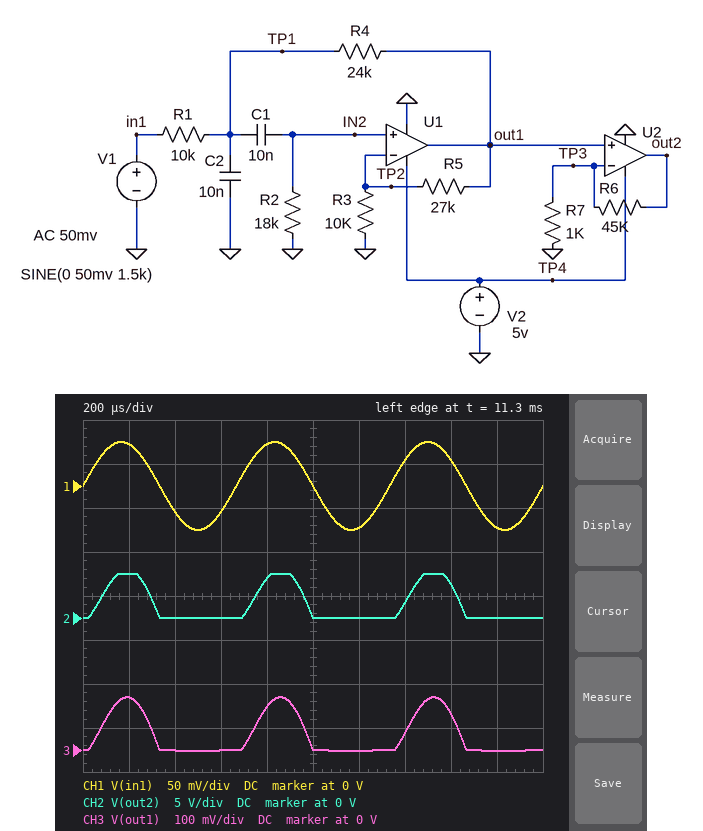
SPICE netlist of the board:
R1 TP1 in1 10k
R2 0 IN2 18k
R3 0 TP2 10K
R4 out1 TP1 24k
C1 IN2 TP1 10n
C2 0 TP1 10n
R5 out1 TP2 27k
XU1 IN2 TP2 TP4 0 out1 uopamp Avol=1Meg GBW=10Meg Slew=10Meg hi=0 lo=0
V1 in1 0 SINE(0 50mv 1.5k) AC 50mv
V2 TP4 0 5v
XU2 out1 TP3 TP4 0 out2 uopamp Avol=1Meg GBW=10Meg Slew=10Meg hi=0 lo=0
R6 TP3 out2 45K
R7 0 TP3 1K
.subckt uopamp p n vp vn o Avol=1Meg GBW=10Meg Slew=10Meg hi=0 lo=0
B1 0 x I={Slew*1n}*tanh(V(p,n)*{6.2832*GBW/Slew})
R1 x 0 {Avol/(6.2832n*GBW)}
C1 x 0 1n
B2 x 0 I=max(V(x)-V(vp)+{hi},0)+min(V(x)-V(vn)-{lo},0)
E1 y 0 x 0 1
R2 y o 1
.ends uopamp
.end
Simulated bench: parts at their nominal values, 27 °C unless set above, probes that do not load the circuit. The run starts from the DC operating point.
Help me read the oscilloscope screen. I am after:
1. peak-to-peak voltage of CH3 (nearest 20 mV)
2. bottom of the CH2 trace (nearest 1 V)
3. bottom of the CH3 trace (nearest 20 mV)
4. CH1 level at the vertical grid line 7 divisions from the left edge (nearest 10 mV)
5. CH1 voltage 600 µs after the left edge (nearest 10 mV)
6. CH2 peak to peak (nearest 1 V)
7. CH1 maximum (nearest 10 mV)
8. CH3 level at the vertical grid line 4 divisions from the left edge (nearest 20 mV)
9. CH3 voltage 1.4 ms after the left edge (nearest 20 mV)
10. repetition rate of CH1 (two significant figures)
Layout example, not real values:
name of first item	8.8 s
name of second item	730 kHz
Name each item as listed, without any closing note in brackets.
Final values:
peak-to-peak voltage of CH3	120 mV
bottom of the CH2 trace	0 V
bottom of the CH3 trace	0 V
CH1 level at the vertical grid line 7 divisions from the left edge	30 mV
CH1 voltage 600 µs after the left edge	-30 mV
CH2 peak to peak	5 V
CH1 maximum	50 mV
CH3 level at the vertical grid line 4 divisions from the left edge	100 mV
CH3 voltage 1.4 ms after the left edge	40 mV
repetition rate of CH1	1.5 kHz
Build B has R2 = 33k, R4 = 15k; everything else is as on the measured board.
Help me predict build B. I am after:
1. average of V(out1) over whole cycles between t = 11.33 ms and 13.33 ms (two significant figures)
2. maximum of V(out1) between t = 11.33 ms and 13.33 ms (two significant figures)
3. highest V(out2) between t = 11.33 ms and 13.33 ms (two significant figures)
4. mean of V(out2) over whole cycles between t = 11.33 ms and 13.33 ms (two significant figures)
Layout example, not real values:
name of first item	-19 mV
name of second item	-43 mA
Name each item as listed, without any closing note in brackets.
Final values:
average of V(out1) over whole cycles between t = 11.33 ms and 13.33 ms	51 mV
maximum of V(out1) between t = 11.33 ms and 13.33 ms	190 mV
highest V(out2) between t = 11.33 ms and 13.33 ms	5.0 V
mean of V(out2) over whole cycles between t = 11.33 ms and 13.33 ms	1.8 V
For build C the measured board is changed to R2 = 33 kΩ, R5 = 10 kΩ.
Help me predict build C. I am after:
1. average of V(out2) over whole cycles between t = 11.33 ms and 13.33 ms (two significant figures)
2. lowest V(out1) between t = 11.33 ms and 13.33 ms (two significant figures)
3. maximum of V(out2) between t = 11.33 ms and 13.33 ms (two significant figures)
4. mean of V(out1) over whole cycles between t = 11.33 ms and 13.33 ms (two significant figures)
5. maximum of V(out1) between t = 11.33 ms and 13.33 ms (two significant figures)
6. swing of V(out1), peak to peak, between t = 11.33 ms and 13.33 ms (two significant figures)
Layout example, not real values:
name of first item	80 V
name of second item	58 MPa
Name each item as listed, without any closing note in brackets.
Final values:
average of V(out2) over whole cycles between t = 11.33 ms and 13.33 ms	880 mV
lowest V(out1) between t = 11.33 ms and 13.33 ms	-1.7 mV
maximum of V(out2) between t = 11.33 ms and 13.33 ms	2.9 V
mean of V(out1) over whole cycles between t = 11.33 ms and 13.33 ms	19 mV
maximum of V(out1) between t = 11.33 ms and 13.33 ms	63 mV
swing of V(out1), peak to peak, between t = 11.33 ms and 13.33 ms	65 mV
